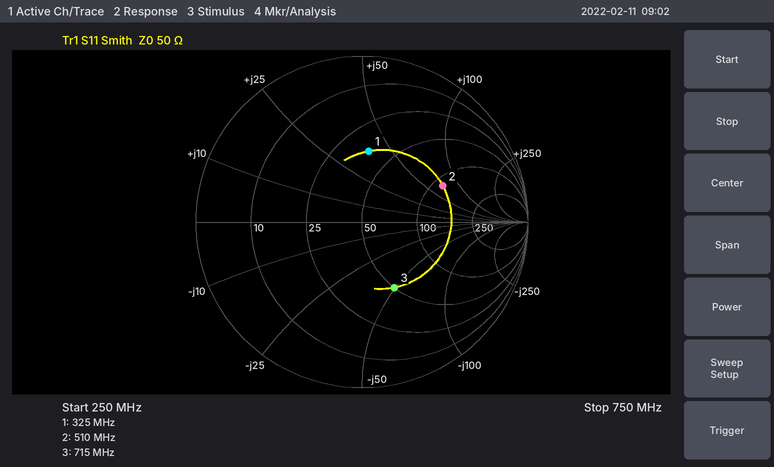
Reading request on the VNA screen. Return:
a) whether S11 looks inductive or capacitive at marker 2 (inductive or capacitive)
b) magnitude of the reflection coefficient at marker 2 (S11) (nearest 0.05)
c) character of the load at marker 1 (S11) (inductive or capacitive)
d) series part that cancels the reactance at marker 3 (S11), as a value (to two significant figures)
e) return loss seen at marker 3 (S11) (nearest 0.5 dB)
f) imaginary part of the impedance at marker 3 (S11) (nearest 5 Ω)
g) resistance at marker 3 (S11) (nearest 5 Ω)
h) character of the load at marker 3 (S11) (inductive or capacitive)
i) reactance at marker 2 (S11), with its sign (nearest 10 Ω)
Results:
inductive
0.55
inductive
11 nH
7.0 dB
-50 Ω
50 Ω
capacitive
+70 Ω
